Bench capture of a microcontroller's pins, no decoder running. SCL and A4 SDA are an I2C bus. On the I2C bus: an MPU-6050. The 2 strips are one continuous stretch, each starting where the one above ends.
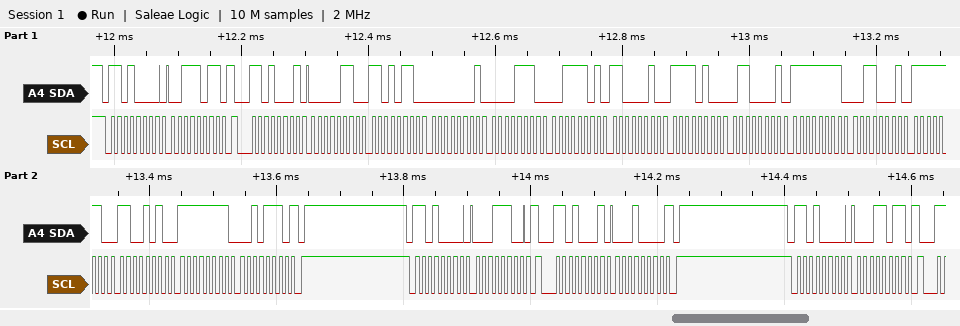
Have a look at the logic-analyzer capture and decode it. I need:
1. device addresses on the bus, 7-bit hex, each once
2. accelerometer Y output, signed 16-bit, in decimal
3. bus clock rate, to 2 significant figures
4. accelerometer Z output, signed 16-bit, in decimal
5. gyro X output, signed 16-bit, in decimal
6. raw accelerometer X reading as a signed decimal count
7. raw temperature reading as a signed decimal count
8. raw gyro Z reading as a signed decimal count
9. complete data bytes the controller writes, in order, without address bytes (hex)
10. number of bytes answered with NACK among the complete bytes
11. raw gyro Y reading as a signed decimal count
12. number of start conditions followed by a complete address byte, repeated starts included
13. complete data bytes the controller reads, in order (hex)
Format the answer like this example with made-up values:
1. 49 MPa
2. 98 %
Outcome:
1. 0x68
2. 270
3. 100 kHz
4. 15810
5. -207
6. 1750
7. -2975
8. -210
9. 3B 1C 1B
10. 2
11. -310
12. 5
13. 06 D6 01 0E 3D C2 F4 61 FF 31 FE CA FF 2E 10
